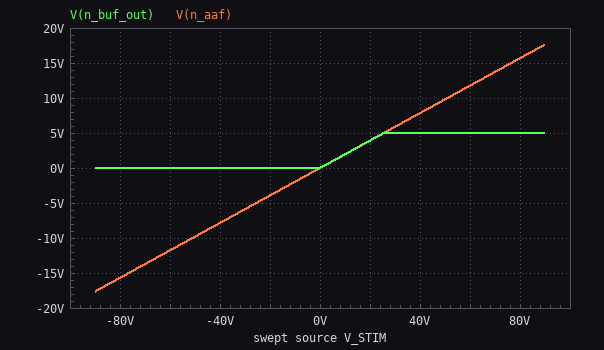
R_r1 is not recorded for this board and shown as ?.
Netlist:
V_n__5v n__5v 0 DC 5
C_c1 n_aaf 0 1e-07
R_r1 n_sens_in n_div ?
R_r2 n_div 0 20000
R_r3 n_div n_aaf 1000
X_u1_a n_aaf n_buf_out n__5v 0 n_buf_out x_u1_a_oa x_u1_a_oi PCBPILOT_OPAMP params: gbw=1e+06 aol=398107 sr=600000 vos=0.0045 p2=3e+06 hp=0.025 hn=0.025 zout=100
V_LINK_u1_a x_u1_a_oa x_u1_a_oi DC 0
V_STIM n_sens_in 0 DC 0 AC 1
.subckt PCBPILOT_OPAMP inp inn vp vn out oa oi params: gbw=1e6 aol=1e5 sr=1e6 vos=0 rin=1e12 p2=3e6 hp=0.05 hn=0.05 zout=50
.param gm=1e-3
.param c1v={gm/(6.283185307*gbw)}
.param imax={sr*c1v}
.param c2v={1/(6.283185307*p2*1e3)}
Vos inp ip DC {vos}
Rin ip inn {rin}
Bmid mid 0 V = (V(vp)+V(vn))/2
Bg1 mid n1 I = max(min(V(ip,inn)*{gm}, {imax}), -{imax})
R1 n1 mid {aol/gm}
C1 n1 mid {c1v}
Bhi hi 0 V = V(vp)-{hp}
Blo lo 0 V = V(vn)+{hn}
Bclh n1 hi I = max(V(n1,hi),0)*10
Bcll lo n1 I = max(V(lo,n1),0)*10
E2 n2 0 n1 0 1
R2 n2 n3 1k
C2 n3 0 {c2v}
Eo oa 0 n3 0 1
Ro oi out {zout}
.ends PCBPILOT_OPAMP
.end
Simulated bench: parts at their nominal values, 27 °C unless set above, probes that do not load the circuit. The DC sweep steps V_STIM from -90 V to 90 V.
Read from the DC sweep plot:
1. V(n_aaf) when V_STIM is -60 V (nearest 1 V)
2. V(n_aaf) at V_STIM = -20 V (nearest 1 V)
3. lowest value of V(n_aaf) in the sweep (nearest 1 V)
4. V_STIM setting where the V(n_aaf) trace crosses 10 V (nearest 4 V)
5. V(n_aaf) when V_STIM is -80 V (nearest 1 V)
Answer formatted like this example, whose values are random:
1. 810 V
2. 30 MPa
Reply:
1. -12 V
2. -4 V
3. -18 V
4. 52 V
5. -16 V
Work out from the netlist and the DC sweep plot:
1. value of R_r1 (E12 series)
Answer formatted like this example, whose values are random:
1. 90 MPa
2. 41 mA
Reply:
1. 82 kΩ
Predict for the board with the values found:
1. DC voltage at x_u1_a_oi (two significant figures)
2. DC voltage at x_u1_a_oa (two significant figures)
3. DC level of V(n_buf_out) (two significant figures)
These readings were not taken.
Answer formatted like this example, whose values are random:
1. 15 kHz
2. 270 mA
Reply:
1. 25 mV
2. 25 mV
3. 25 mV
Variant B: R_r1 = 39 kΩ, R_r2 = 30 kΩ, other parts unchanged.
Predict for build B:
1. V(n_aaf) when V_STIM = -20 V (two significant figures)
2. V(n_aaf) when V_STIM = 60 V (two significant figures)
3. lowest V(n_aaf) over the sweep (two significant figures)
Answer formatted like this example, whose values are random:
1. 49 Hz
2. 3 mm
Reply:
1. -8.7 V
2. 26 V
3. -39 V
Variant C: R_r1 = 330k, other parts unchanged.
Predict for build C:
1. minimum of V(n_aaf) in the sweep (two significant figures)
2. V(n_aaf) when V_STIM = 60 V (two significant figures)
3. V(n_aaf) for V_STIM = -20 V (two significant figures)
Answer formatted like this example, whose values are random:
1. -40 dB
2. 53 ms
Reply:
1. -5.1 V
2. 3.4 V
3. -1.1 V
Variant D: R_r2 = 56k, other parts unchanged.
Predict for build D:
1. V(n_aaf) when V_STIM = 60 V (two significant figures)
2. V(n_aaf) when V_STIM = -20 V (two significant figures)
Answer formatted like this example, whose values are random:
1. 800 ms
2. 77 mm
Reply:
1. 24 V
2. -8.1 V
